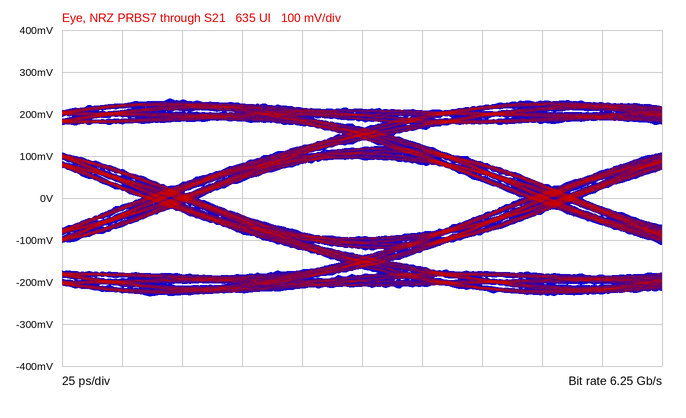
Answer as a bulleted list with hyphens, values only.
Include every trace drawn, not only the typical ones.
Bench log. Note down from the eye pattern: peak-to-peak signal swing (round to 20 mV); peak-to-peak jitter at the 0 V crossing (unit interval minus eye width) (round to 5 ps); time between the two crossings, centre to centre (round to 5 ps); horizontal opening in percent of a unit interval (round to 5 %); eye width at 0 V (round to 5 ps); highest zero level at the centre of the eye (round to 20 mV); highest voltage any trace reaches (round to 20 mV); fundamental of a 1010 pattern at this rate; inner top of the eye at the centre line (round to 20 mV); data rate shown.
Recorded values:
- 460 mV
- 25 ps
- 160 ps
- 85 %
- 135 ps
- -100 mV
- 240 mV
- 3.125 GHz
- 100 mV
- 6.25 Gb/s
